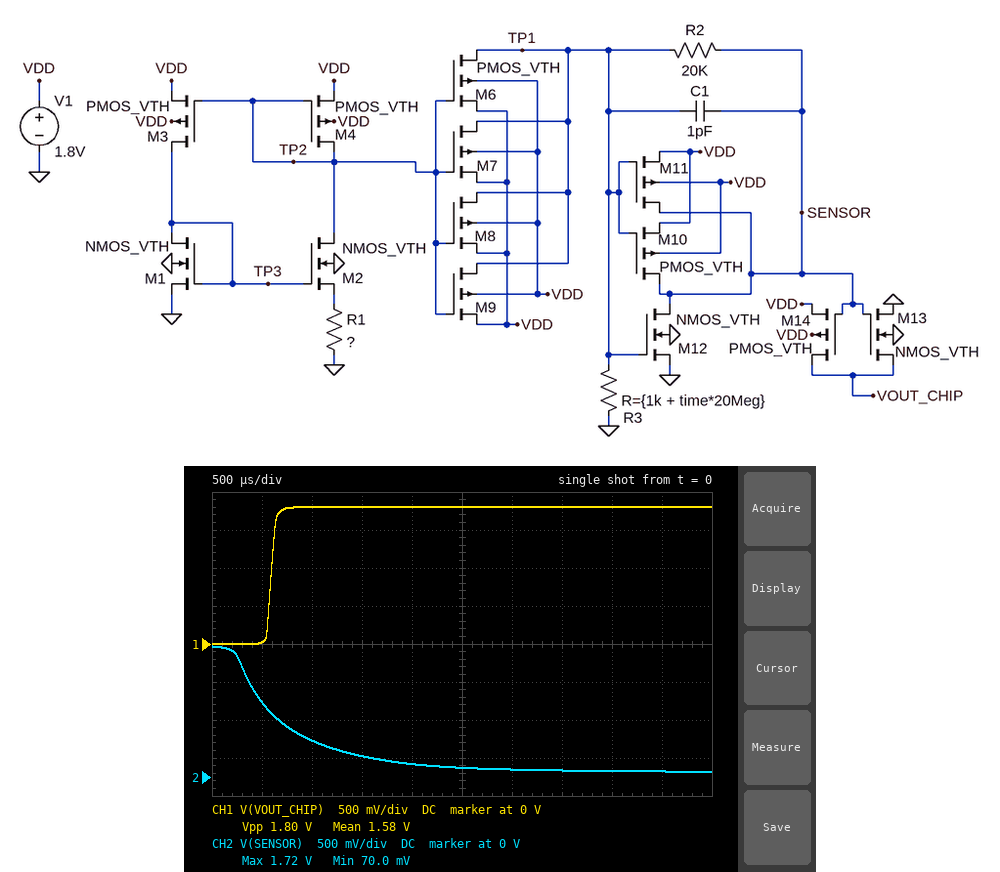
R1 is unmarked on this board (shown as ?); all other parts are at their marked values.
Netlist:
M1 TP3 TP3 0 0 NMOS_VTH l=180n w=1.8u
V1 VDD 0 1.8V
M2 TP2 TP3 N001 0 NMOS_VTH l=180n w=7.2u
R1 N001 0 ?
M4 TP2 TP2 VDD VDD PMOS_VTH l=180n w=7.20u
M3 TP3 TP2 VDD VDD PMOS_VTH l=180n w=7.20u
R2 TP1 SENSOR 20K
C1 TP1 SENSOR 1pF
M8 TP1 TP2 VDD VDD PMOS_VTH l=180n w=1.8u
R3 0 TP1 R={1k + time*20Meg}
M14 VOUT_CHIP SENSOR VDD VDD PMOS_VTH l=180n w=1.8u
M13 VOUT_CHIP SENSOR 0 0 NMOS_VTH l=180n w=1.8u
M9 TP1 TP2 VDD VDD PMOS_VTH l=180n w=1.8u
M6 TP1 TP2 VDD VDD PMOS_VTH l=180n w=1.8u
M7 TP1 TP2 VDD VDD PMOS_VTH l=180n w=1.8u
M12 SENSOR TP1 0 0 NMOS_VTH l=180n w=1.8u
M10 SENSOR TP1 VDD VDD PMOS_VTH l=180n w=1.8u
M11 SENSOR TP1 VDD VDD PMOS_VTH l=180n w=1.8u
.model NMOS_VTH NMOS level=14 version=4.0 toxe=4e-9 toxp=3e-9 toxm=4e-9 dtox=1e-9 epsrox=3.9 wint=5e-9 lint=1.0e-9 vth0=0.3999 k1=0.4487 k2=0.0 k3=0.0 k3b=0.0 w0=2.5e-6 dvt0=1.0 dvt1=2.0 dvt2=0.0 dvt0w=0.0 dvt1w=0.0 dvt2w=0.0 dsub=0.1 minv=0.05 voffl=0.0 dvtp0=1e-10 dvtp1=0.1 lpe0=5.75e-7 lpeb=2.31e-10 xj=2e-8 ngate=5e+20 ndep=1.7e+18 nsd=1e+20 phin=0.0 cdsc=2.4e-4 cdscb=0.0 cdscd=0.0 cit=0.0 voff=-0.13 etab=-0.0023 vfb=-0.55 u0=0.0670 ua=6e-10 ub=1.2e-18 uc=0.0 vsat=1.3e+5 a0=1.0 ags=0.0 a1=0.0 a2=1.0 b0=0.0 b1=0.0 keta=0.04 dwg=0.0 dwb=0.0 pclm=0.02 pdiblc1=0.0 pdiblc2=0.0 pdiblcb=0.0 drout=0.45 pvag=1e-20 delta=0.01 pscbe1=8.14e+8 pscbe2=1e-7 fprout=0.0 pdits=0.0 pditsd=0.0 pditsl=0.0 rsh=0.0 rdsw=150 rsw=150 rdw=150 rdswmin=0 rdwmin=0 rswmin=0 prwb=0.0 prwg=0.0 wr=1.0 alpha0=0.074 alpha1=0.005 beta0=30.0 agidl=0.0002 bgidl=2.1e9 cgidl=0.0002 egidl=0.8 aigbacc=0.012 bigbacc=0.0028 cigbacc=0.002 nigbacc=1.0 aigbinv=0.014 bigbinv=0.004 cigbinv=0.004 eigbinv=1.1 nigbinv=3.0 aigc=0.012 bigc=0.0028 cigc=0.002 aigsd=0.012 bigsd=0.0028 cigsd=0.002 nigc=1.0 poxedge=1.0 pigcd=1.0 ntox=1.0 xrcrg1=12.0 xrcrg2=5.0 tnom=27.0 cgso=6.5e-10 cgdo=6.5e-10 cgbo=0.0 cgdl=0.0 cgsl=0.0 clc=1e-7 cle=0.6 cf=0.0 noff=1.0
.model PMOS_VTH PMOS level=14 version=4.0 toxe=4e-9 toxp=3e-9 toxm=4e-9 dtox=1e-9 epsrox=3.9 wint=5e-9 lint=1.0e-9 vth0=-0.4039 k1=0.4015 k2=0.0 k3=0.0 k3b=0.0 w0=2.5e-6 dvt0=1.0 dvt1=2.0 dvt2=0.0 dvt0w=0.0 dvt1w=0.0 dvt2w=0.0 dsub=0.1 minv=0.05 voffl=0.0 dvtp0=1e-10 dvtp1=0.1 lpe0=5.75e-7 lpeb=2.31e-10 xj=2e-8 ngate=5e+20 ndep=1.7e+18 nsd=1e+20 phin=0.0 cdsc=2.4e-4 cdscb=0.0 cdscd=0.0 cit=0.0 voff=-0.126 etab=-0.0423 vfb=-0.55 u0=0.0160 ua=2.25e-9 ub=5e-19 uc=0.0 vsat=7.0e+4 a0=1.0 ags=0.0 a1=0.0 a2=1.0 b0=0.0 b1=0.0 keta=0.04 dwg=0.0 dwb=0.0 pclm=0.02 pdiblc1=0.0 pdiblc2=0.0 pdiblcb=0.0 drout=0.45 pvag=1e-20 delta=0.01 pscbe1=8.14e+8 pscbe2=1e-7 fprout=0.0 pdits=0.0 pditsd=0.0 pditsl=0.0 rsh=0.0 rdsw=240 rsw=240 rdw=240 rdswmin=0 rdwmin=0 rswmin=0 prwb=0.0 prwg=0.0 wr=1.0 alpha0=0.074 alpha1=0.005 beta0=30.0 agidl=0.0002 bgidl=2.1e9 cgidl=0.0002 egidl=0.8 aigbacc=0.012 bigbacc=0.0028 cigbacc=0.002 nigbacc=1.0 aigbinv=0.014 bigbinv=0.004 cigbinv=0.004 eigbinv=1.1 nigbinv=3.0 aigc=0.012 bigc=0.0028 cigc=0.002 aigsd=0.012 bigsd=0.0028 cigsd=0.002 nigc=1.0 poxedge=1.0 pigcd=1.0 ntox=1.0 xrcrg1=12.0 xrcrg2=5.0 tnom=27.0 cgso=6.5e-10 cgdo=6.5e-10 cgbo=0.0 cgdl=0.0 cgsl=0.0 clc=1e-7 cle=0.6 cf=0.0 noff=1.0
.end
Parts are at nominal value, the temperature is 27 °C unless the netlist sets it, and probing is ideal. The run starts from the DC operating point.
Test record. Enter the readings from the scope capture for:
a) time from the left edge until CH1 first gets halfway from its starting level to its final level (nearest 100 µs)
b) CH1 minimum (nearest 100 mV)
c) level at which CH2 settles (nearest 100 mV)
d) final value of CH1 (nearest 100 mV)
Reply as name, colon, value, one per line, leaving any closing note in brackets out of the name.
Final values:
time from the left edge until CH1 first gets halfway from its starting level to its final level: 600 µs
CH1 minimum: 0 V
level at which CH2 settles: 100 mV
final value of CH1: 1.8 V
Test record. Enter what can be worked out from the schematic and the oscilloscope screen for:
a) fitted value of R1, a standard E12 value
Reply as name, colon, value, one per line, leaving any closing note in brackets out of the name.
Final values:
fitted value of R1, a standard E12 value: 1.2 kΩ
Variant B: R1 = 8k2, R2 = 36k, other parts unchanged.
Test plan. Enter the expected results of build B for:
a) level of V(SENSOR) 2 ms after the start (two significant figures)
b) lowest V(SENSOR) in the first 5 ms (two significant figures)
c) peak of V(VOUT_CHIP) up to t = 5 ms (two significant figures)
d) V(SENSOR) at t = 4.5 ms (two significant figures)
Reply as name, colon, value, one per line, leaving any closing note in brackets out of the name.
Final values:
level of V(SENSOR) 2 ms after the start: 1.1 V
lowest V(SENSOR) in the first 5 ms: 790 mV
peak of V(VOUT_CHIP) up to t = 5 ms: 1.6 V
V(SENSOR) at t = 4.5 ms: 820 mV
